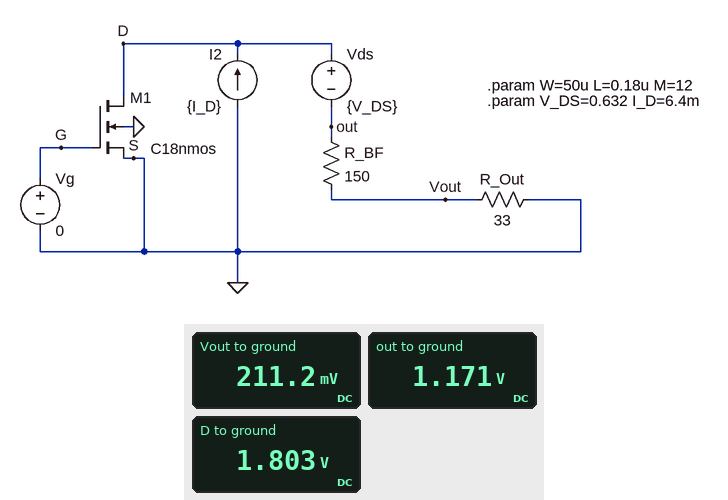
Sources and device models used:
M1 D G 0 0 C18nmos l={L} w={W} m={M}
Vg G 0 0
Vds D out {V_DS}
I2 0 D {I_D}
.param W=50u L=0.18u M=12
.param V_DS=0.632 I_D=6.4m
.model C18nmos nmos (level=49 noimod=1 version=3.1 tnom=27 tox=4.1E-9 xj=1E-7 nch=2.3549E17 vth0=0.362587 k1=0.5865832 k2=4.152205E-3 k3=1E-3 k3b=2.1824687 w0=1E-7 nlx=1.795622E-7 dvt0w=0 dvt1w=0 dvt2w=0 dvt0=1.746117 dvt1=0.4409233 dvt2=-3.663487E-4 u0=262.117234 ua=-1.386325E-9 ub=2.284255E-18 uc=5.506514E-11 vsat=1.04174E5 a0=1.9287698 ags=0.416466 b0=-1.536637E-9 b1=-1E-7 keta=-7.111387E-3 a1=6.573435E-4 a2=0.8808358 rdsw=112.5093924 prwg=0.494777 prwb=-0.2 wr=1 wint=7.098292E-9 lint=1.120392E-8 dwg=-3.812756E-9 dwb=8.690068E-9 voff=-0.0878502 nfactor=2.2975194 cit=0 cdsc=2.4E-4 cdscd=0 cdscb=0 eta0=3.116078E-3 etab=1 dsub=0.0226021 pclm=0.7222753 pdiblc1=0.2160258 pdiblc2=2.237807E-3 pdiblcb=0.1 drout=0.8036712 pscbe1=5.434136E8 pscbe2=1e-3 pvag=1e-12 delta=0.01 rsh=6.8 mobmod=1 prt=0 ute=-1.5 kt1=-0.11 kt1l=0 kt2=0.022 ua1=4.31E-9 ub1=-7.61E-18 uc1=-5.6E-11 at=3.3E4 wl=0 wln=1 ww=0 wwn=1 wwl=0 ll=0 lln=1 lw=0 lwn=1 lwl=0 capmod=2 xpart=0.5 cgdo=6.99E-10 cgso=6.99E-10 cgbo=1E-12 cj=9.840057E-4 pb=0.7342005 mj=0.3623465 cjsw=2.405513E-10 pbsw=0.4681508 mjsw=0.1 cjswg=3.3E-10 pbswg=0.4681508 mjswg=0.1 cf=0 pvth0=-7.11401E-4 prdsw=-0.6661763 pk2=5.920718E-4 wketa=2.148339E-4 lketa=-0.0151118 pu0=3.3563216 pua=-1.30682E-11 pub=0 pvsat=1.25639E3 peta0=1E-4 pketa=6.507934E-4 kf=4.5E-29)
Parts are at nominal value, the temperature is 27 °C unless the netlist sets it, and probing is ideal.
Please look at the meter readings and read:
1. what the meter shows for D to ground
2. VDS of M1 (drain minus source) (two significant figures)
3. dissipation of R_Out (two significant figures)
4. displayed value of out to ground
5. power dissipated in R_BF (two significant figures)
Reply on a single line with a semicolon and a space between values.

1.803 V; 1.8 V; 1.4 mW; 1.171 V; 6.1 mW
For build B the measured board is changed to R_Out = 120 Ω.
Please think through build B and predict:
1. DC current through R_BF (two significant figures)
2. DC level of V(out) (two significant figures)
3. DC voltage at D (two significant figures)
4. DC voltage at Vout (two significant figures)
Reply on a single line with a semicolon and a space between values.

6.4 mA; 1.7 V; 2.4 V; 770 mV
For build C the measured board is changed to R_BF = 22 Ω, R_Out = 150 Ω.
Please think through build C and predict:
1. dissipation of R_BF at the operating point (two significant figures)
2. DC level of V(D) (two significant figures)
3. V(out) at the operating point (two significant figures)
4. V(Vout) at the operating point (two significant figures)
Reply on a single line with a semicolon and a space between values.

900 µW; 1.7 V; 1.1 V; 960 mV
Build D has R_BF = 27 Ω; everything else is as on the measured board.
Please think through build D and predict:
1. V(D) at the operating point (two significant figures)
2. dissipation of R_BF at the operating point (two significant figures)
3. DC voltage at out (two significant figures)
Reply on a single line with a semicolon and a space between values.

1.0 V; 1.1 mW; 380 mV
